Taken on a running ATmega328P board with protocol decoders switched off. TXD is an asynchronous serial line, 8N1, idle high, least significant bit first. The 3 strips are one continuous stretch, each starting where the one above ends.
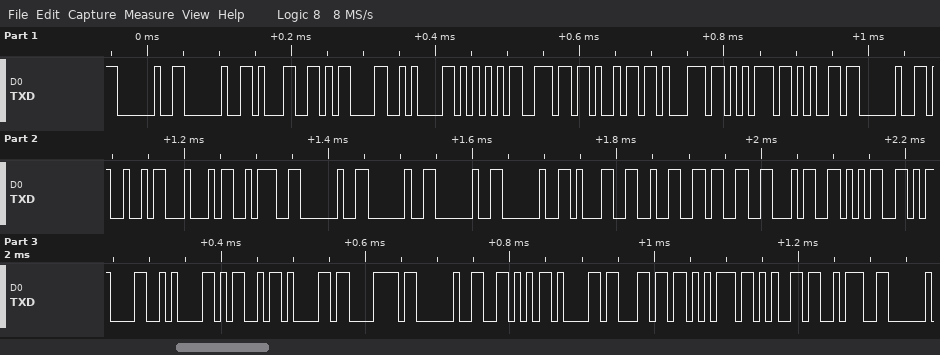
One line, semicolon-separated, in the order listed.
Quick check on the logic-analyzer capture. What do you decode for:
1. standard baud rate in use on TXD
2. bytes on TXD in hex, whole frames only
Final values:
115200 baud; 0x20 0x20 0x31 0x0D 0x0A 0x55 0x6E 0x69 0x71 0x75 0x65 0x20 0x49 0x44 0x3A 0x20 0x20 0x20 0x20 0x31 0x32 0x33 0x34 0x35 0x0D 0x0A 0x4D 0x61 0x78 0x20 0x56 0x61 0x6C 0x75 0x65 0x3A
